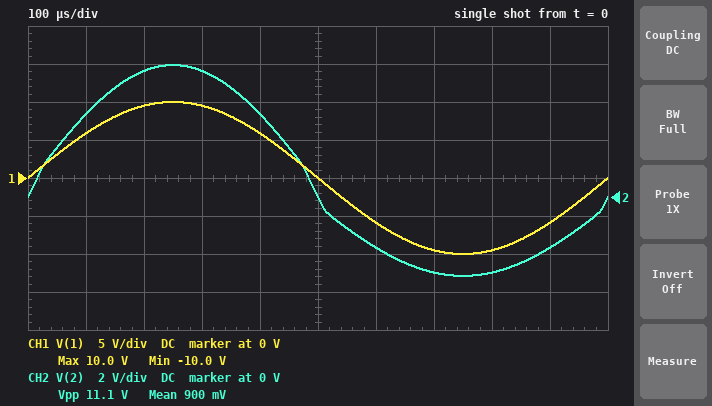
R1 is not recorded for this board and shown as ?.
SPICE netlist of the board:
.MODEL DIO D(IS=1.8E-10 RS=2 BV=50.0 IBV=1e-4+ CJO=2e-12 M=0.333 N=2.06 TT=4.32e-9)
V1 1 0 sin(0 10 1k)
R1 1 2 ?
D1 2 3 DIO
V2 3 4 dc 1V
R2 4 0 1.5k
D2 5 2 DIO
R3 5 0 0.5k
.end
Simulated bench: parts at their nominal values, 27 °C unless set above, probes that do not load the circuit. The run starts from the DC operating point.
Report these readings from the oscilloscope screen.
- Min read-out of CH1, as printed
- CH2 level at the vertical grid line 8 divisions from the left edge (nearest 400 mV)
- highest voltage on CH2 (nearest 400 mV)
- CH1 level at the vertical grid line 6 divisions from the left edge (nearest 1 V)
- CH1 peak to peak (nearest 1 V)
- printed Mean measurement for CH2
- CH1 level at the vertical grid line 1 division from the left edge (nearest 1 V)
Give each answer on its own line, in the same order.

-10.0 V
-4.0 V
6.8 V
-6 V
20 V
900 mV
6 V
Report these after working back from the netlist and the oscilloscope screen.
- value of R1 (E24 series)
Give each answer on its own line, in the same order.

910 Ω
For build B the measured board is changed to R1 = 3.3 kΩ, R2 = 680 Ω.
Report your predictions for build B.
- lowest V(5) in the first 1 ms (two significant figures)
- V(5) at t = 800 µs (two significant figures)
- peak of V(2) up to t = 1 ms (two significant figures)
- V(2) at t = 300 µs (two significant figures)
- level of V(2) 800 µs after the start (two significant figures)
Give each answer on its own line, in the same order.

-1.2 V
-1.1 V
3.3 V
3.2 V
-2.0 V
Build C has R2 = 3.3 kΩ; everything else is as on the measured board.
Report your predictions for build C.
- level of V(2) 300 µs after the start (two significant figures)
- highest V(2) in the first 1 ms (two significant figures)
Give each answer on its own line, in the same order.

7.9 V
8.2 V
